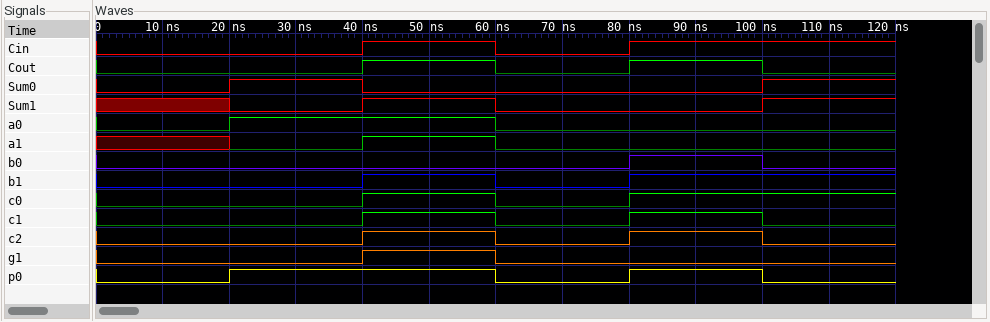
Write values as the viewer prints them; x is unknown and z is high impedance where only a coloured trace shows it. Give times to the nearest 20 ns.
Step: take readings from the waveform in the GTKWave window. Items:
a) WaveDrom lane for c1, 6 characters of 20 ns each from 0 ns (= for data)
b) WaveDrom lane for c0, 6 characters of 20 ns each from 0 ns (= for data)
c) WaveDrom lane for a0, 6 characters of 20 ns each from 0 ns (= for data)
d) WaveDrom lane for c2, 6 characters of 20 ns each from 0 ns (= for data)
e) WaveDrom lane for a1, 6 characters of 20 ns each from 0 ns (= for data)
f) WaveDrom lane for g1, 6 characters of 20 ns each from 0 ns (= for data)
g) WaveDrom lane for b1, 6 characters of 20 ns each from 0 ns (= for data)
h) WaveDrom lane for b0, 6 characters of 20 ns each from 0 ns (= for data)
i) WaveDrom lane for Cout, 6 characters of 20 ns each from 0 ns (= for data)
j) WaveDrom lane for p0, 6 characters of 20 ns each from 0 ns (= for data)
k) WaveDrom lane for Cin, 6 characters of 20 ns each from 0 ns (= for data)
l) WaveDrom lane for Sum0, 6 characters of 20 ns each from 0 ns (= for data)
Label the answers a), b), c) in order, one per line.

a) {name: 'c1', wave: '0.1010'}
b) {name: 'c0', wave: '0.101.'}
c) {name: 'a0', wave: '01.0..'}
d) {name: 'c2', wave: '0.1010'}
e) {name: 'a1', wave: 'x010..'}
f) {name: 'g1', wave: '0.10..'}
g) {name: 'b1', wave: '0.101.'}
h) {name: 'b0', wave: '0...10'}
i) {name: 'Cout', wave: '0.1010'}
j) {name: 'p0', wave: '01.010'}
k) {name: 'Cin', wave: '0.101.'}
l) {name: 'Sum0', wave: '010..1'}
